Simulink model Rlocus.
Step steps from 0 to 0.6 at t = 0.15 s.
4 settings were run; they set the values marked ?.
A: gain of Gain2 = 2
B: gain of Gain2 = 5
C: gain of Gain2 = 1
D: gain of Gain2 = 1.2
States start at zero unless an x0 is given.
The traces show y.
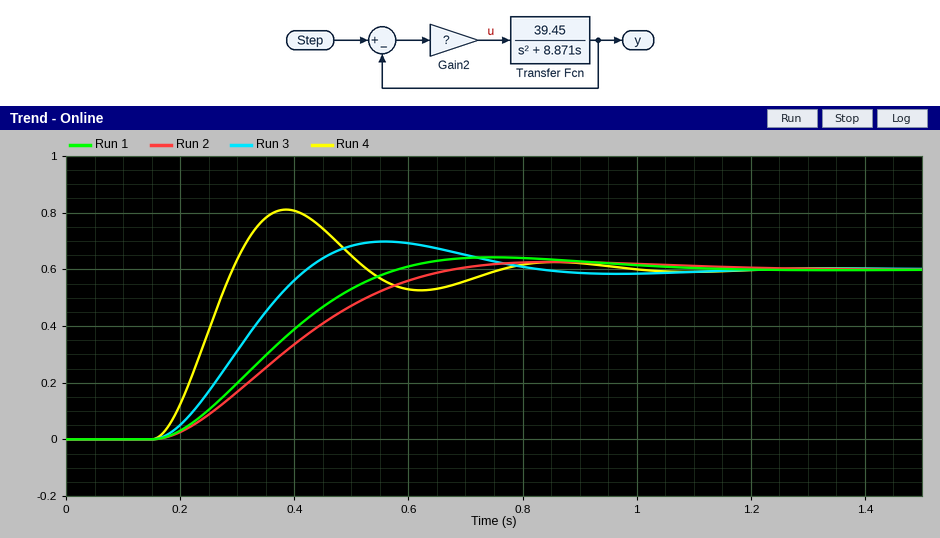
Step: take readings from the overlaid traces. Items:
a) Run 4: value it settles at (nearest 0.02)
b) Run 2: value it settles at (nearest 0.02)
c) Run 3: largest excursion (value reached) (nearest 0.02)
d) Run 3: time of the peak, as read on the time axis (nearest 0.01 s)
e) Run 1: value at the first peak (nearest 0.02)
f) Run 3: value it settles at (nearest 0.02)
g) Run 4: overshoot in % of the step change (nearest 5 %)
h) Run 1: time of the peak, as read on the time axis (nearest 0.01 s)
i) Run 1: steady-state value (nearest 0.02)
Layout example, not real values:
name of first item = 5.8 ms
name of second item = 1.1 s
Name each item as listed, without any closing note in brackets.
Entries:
Run 4: value it settles at = 0.60
Run 2: value it settles at = 0.60
Run 3: largest excursion (value reached) = 0.70
Run 3: time of the peak, as read on the time axis = 0.56 s
Run 1: value at the first peak = 0.64
Run 3: value it settles at = 0.60
Run 4: overshoot in % of the step change = 35 %
Run 1: time of the peak, as read on the time axis = 0.75 s
Run 1: steady-state value = 0.60
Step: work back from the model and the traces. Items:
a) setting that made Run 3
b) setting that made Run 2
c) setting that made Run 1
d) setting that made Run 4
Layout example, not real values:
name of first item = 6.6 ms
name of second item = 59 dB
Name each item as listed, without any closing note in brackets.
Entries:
setting that made Run 3 = A
setting that made Run 2 = C
setting that made Run 1 = D
setting that made Run 4 = B
